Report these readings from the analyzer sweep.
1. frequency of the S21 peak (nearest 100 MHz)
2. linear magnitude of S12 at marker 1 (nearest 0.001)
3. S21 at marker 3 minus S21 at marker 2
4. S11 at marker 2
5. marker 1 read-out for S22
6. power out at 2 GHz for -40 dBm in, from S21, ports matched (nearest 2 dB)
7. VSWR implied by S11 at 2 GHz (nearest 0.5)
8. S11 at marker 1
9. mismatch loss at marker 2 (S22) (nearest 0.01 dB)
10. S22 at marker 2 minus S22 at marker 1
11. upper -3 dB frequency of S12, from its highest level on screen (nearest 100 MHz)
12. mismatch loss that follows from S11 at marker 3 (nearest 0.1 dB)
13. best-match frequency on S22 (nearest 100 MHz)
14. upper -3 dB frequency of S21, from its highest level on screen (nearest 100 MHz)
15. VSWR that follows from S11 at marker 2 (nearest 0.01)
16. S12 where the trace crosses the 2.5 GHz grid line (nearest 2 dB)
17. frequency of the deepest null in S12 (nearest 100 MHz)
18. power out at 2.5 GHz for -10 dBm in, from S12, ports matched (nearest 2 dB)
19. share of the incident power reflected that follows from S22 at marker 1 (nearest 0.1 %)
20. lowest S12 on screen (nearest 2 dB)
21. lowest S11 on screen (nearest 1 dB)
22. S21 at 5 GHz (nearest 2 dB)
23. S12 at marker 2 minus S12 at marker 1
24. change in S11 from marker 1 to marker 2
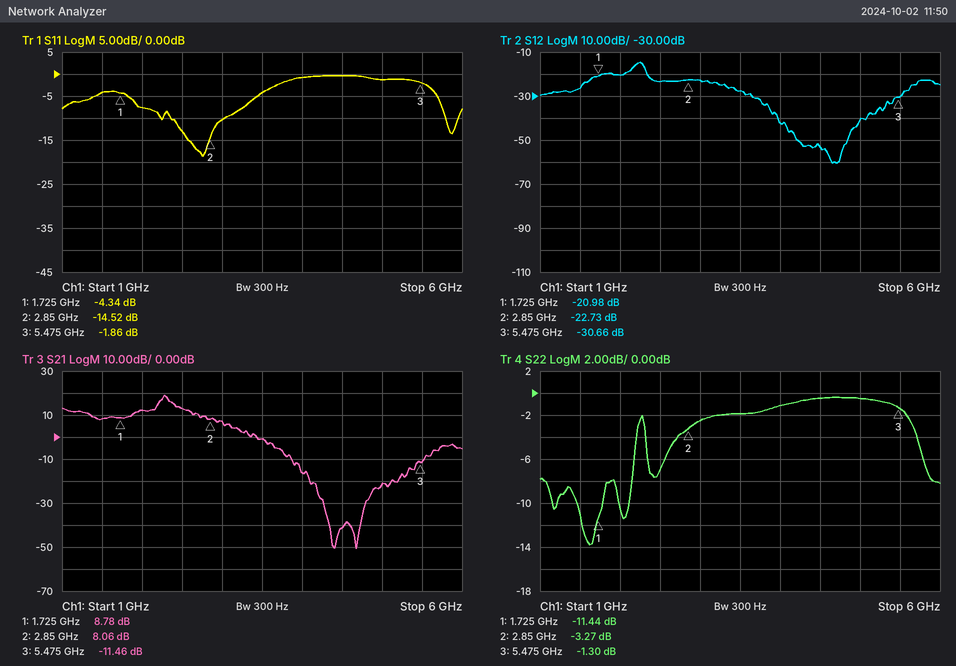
2.3 GHz
0.089
-19.52 dB
-14.52 dB
-11.44 dB
-28 dBm
2.5
-4.34 dB
2.77 dB
8.17 dB
2.3 GHz
4.6 dB
1.6 GHz
2.4 GHz
1.46
-24 dB
4.7 GHz
-34 dBm
7.2 %
-60 dB
-19 dB
-22 dB
-1.75 dB
-10.18 dB
